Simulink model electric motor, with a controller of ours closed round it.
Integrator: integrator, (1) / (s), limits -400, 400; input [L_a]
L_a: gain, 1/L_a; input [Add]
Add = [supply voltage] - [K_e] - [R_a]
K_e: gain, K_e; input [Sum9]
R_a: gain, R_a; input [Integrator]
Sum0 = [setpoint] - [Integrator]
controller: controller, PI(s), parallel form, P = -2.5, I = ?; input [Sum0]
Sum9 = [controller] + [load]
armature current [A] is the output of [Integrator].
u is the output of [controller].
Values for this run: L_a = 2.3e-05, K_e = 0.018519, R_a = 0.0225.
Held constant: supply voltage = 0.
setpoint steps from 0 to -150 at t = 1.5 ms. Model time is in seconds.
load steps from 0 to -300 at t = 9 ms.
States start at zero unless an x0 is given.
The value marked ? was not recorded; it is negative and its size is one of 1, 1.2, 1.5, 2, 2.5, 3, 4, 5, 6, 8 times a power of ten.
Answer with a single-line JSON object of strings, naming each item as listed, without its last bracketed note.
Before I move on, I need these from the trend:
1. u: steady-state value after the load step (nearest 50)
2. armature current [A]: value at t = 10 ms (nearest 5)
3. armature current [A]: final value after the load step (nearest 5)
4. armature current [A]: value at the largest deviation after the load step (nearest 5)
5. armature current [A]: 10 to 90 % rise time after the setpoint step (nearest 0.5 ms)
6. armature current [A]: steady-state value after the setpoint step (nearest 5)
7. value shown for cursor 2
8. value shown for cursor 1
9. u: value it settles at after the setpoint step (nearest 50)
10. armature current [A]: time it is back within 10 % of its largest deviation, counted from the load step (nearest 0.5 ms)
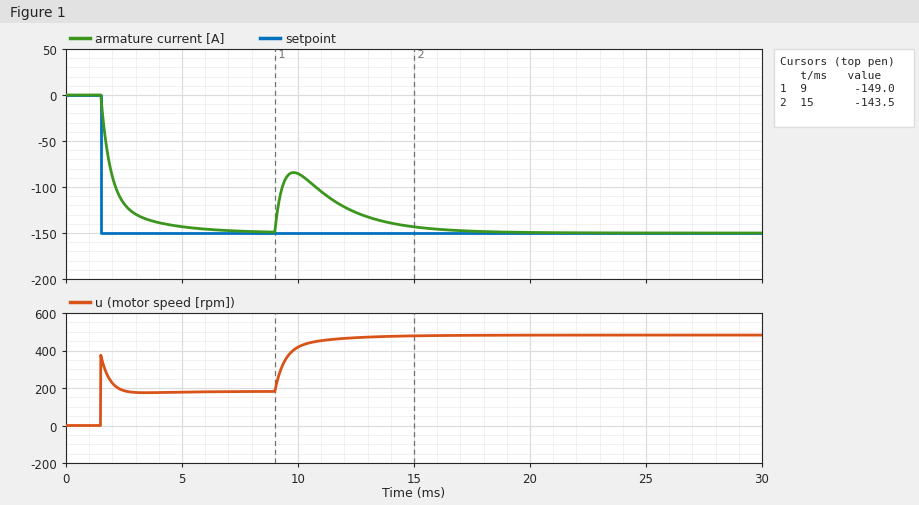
{"u: steady-state value after the load step": "500", "armature current [A]: value at t = 10 ms": "-85", "armature current [A]: final value after the load step": "-150", "armature current [A]: value at the largest deviation after the load step": "-85", "armature current [A]: 10 to 90 % rise time after the setpoint step": "2.0 ms", "armature current [A]: steady-state value after the setpoint step": "-150", "value shown for cursor 2": "-143.5", "value shown for cursor 1": "-149.0", "u: value it settles at after the setpoint step": "200", "armature current [A]: time it is back within 10 % of its largest deviation, counted from the load step": "6.0 ms"}
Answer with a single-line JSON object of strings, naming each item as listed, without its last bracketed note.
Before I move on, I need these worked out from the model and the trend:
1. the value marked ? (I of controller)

{"the value marked ?": "-1500"}
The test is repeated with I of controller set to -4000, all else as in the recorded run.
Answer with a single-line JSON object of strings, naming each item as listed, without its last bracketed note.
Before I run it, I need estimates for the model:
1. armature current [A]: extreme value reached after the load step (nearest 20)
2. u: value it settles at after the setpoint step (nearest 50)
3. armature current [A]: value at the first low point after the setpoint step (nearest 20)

{"armature current [A]: extreme value reached after the load step": "-100", "u: value it settles at after the setpoint step": "200", "armature current [A]: value at the first low point after the setpoint step": "-160"}
